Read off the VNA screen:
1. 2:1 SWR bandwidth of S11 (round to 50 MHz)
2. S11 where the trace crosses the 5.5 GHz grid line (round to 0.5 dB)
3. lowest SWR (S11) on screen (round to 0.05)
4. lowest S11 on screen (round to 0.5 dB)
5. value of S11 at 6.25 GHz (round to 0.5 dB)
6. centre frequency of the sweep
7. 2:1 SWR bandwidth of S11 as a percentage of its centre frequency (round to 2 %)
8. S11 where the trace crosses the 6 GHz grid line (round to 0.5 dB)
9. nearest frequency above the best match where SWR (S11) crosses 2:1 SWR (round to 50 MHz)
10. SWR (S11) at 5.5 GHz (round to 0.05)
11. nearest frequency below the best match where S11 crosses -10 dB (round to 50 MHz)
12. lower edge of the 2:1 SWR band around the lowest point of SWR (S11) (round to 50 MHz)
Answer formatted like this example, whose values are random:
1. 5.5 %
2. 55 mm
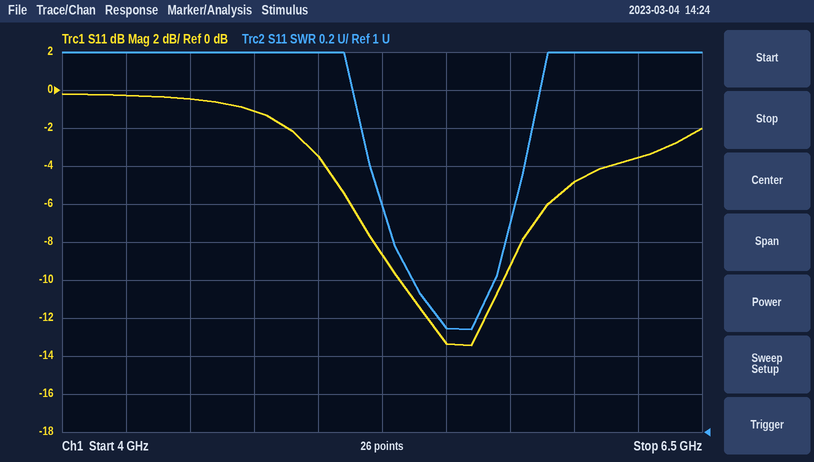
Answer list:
1. 450 MHz
2. -13.5 dB
3. 1.55
4. -13.5 dB
5. -3.5 dB
6. 5.25 GHz
7. 8 %
8. -5.0 dB
9. 5.75 GHz
10. 1.55
11. 5.30 GHz
12. 5.30 GHz
